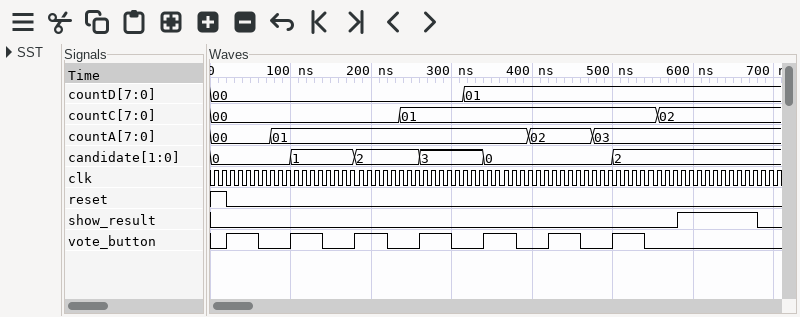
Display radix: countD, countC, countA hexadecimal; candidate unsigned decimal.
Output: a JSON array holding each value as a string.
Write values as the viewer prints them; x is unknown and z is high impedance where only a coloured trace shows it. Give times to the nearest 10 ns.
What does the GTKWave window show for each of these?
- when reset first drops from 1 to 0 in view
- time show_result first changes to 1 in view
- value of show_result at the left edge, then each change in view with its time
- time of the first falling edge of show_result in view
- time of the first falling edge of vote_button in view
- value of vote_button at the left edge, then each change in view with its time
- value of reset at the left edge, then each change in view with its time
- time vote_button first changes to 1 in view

["20 ns", "580 ns", "0, 1 at 580 ns, 0 at 680 ns", "680 ns", "60 ns", "0, 1 at 20 ns, 0 at 60 ns, 1 at 100 ns, 0 at 140 ns, 1 at 180 ns, 0 at 220 ns, 1 at 260 ns, 0 at 300 ns, 1 at 340 ns, 0 at 380 ns, 1 at 420 ns, 0 at 460 ns, 1 at 500 ns, 0 at 540 ns", "1, 0 at 20 ns", "20 ns"]
